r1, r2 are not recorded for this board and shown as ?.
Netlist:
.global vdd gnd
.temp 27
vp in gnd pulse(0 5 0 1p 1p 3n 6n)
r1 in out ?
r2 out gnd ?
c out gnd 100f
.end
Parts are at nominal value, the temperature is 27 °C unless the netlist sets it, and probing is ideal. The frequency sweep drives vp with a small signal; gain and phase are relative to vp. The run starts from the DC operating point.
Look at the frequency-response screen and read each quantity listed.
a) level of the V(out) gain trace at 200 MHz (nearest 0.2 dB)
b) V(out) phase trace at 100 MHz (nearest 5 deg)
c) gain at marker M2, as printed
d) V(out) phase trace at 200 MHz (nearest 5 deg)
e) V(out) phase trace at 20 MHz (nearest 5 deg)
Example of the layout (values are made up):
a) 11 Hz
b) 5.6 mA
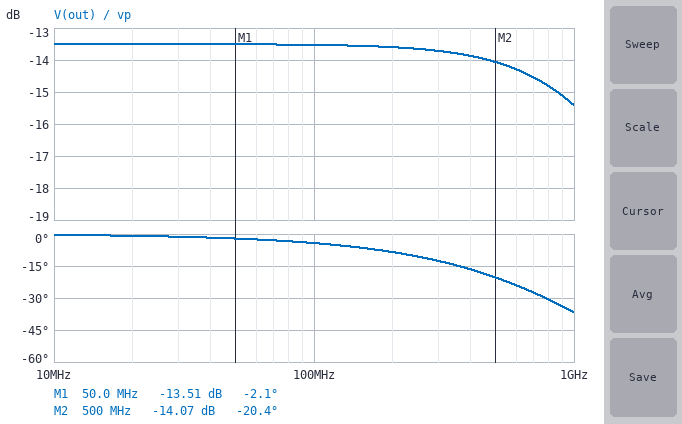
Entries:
a) -13.6 dB
b) -5 deg
c) -14.07 dB
d) -10 deg
e) 0 deg
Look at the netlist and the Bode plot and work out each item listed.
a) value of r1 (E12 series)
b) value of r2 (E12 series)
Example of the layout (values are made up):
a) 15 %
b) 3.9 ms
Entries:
a) 5.6 kΩ
b) 1.5 kΩ
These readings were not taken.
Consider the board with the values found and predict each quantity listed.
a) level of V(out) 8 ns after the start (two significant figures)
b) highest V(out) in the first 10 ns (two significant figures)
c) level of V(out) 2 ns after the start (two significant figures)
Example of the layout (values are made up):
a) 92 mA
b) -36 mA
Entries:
a) 1.1 V
b) 1.1 V
c) 1.1 V
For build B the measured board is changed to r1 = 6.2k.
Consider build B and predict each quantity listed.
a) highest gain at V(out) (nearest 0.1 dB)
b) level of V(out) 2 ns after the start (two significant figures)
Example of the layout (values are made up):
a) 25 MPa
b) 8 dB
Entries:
a) -14.2 dB
b) 970 mV
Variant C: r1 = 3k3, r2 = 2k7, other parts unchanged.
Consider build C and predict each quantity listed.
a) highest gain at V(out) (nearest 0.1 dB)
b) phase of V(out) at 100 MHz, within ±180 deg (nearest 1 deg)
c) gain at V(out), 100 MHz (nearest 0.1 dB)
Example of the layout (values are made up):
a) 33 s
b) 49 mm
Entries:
a) -6.9 dB
b) -5 deg
c) -7.0 dB
